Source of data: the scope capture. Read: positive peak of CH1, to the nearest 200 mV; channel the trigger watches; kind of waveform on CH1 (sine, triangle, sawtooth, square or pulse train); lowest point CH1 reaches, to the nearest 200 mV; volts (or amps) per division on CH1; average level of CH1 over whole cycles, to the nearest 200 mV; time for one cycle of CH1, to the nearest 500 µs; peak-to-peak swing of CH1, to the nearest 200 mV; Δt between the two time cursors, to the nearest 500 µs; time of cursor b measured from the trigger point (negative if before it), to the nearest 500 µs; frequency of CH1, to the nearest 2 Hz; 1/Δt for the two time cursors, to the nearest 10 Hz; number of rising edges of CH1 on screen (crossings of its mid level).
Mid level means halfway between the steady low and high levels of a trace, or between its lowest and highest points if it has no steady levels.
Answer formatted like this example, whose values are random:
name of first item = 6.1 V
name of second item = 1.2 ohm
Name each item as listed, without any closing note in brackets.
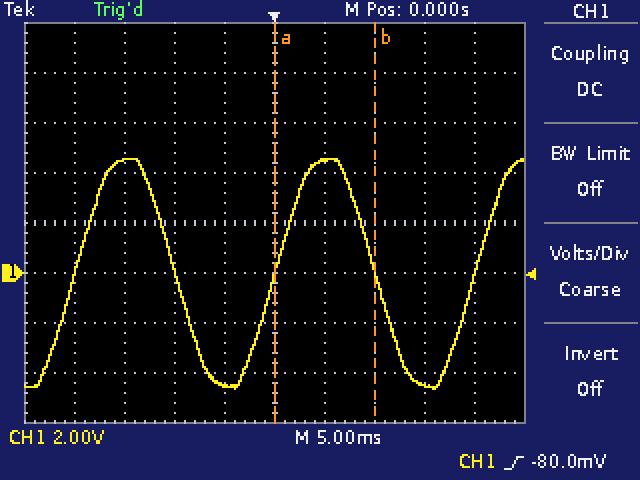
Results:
positive peak of CH1, to the nearest 200 mV = 4.6 V
channel the trigger watches = CH1
kind of waveform on CH1 = sine
lowest point CH1 reaches, to the nearest 200 mV = -4.6 V
volts (or amps) per division on CH1 = 2 V
average level of CH1 over whole cycles, to the nearest 200 mV = 0.0 V
time for one cycle of CH1, to the nearest 500 µs = 20.0 ms
peak-to-peak swing of CH1, to the nearest 200 mV = 9.2 V
Δt between the two time cursors, to the nearest 500 µs = 10.0 ms
time of cursor b measured from the trigger point (negative if before it), to the nearest 500 µs = +10.0 ms
frequency of CH1, to the nearest 2 Hz = 50 Hz
1/Δt for the two time cursors, to the nearest 10 Hz = 100 Hz
number of rising edges of CH1 on screen = 3
